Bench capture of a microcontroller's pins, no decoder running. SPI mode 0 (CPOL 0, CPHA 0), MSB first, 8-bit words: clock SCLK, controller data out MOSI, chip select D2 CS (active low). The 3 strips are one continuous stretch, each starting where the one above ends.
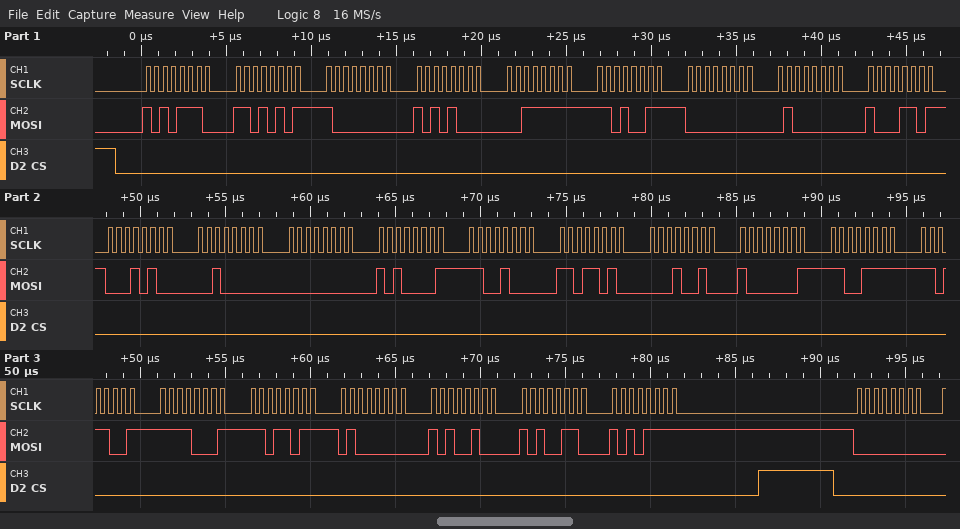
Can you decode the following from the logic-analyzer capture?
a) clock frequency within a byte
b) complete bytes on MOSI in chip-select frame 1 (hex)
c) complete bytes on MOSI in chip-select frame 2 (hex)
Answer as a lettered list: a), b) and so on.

a) 2 MHz
b) AE D5 80 A8 3F D3 00 40 8D 14 20 00 A1 C8 DA 12 81 CF D9 F1 DB 40 A4 A6 AF
c) 00
